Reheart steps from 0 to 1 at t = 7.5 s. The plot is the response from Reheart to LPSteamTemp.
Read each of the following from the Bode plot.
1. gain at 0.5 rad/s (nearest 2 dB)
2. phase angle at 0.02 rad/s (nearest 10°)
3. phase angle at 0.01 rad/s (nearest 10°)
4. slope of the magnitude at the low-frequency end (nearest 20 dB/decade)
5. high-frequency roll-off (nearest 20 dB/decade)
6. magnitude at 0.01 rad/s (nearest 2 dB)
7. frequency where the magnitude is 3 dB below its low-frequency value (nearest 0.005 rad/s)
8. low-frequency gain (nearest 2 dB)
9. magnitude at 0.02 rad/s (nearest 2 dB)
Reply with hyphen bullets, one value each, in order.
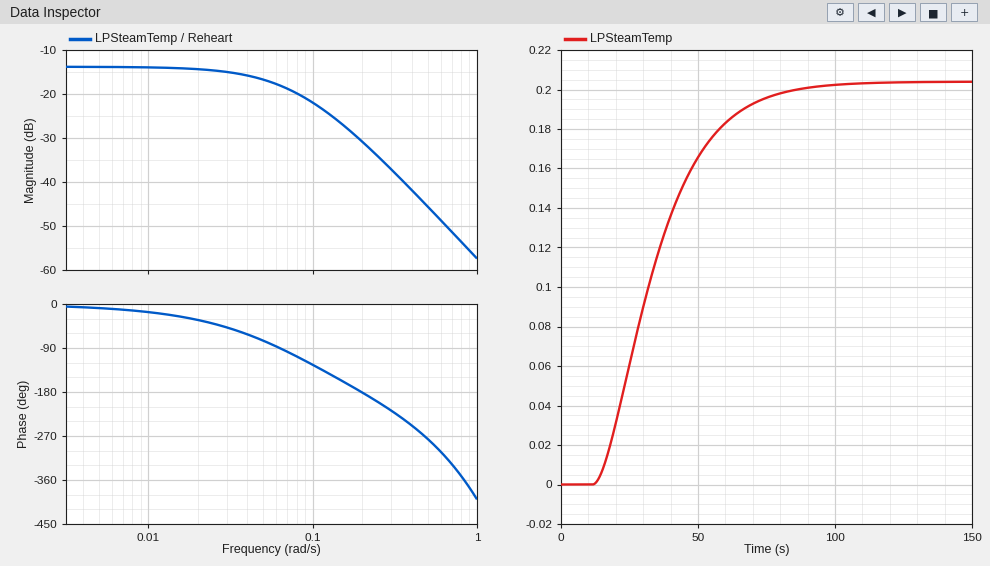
- -46 dB
- -30°
- -20°
- 0 dB/decade
- -40 dB/decade
- -14 dB
- 0.050 rad/s
- -14 dB
- -14 dB
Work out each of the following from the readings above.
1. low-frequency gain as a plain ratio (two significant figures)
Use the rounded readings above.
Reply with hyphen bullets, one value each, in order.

- 0.20
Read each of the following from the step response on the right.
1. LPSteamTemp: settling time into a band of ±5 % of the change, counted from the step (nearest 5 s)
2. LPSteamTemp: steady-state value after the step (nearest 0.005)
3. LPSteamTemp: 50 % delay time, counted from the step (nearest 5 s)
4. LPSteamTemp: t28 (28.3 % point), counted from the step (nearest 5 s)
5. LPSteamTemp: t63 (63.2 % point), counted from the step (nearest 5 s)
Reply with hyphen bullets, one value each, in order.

- 65 s
- 0.205
- 25 s
- 15 s
- 30 s
